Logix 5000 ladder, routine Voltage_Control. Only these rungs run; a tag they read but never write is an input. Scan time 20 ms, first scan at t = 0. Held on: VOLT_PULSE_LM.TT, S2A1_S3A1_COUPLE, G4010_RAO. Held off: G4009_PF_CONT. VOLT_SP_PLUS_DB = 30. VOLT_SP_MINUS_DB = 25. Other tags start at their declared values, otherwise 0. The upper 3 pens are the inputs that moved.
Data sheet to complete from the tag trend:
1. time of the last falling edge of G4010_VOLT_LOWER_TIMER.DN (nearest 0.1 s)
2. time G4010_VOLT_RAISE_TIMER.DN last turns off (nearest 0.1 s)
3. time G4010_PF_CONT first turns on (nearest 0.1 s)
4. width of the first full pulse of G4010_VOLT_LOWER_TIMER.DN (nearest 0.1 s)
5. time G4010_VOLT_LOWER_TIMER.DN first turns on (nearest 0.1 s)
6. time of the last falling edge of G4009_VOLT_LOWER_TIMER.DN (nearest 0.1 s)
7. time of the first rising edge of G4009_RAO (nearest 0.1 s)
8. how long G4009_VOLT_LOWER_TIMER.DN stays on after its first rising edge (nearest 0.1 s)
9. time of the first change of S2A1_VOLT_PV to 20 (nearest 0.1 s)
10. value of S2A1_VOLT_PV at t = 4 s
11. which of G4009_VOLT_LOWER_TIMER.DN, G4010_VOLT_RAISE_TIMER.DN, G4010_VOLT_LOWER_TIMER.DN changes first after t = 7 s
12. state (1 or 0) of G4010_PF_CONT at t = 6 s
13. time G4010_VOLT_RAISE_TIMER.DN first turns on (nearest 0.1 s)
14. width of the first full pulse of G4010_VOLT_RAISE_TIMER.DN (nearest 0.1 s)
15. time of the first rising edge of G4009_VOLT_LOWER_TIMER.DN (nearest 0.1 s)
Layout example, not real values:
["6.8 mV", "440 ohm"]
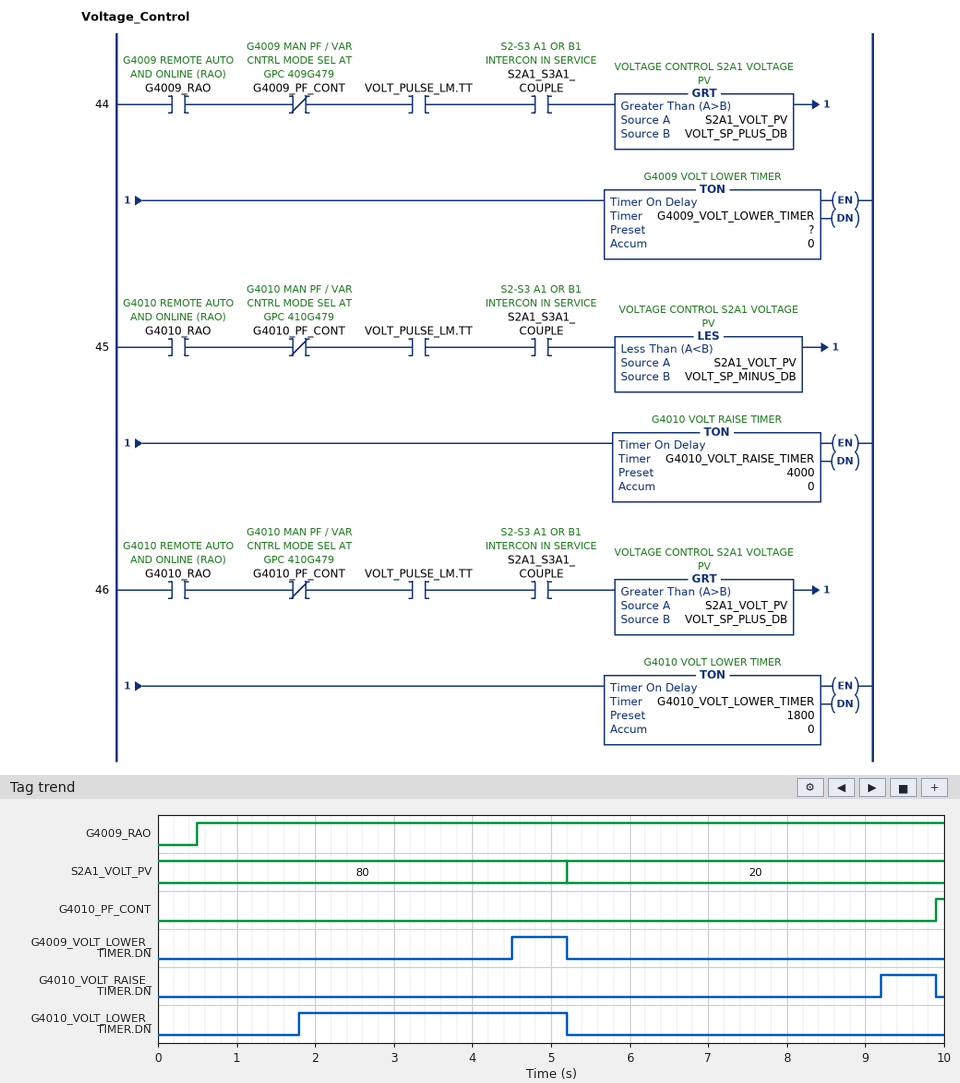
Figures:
["5.2 s", "9.9 s", "9.9 s", "3.4 s", "1.8 s", "5.2 s", "0.5 s", "0.7 s", "5.2 s", "80", "G4010_VOLT_RAISE_TIMER.DN", "0", "9.2 s", "0.7 s", "4.5 s"]
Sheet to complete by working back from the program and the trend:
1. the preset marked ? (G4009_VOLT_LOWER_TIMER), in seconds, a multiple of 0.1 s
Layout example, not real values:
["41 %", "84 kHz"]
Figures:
["4.0 s"]
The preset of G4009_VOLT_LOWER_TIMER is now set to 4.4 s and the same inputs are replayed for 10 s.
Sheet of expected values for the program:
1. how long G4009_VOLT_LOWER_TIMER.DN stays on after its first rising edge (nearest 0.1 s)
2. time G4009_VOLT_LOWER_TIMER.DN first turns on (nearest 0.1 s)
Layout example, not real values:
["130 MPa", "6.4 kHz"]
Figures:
["0.3 s", "4.9 s"]
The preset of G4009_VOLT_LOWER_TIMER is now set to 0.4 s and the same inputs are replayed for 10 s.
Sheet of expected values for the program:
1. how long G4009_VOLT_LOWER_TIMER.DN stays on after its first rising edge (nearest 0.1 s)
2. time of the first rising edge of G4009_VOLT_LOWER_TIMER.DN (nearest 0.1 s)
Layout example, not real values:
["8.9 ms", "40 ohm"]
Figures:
["4.3 s", "0.9 s"]
